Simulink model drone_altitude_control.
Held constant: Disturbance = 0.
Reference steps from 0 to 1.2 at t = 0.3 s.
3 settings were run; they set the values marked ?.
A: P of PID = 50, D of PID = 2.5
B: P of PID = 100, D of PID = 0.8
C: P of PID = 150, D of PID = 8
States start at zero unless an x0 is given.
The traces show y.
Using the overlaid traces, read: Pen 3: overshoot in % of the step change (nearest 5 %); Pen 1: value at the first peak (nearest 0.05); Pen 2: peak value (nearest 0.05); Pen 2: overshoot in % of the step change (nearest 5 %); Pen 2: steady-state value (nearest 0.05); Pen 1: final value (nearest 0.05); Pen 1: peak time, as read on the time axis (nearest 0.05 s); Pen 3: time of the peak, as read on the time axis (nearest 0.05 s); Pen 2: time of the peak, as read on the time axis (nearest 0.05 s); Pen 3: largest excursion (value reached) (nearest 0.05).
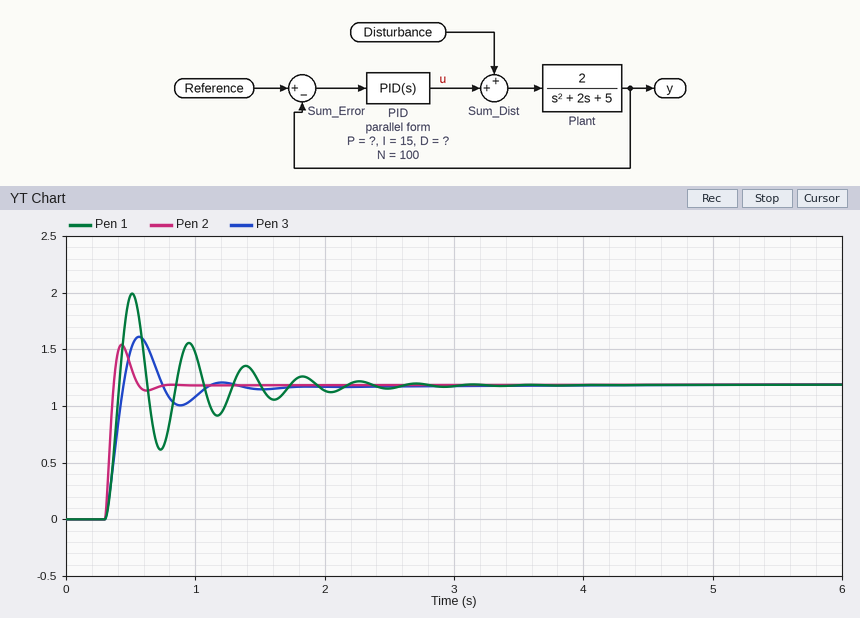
35 %
2.00
1.55
30 %
1.20
1.20
0.50 s
0.55 s
0.45 s
1.60
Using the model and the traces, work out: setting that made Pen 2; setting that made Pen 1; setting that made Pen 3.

C
B
A
